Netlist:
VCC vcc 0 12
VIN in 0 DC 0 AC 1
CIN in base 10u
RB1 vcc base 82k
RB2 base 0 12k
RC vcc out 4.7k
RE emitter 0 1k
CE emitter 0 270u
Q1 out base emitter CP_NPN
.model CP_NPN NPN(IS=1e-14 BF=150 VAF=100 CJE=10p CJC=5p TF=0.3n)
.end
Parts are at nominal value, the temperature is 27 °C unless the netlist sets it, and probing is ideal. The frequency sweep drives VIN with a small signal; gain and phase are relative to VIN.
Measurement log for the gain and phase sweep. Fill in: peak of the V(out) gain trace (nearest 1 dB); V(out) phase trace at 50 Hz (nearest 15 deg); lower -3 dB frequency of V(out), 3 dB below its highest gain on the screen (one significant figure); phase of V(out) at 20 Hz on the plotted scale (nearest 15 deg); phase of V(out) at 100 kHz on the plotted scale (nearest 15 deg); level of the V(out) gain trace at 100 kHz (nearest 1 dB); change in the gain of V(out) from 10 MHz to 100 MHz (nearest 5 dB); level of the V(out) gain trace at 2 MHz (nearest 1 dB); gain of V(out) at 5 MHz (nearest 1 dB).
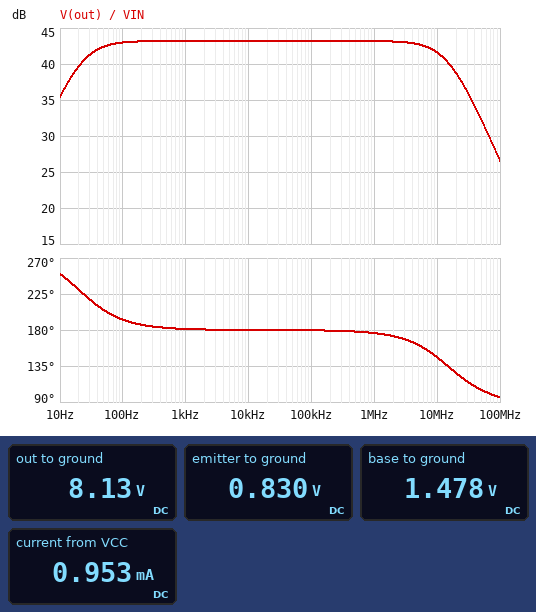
43 dB
210 deg
20 Hz
225 deg
180 deg
43 dB
-15 dB
43 dB
43 dB
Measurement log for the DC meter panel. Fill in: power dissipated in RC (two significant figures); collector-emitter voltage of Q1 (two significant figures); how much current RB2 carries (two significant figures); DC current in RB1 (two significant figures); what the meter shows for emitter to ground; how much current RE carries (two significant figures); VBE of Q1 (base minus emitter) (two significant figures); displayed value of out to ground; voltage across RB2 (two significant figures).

3.2 mW
7.3 V
120 µA
130 µA
0.830 V
830 µA
650 mV
8.13 V
1.5 V
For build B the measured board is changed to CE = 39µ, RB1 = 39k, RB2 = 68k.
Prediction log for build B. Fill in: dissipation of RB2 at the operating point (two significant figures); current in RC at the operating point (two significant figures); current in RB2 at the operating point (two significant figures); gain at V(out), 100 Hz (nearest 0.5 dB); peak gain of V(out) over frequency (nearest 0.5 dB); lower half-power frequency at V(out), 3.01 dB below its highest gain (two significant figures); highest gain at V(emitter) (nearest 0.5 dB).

130 µW
2.1 mA
43 µA
-4.0 dB
15.5 dB
940 Hz
-13.5 dB
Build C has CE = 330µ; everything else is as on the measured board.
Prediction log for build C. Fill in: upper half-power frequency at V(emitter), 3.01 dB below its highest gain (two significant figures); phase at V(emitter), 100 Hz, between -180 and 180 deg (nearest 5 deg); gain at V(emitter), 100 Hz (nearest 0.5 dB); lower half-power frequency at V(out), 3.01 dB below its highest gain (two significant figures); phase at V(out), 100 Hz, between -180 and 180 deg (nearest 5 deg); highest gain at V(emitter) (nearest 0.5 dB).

21 Hz
-80 deg
-16.5 dB
19 Hz
-170 deg
-2.5 dB
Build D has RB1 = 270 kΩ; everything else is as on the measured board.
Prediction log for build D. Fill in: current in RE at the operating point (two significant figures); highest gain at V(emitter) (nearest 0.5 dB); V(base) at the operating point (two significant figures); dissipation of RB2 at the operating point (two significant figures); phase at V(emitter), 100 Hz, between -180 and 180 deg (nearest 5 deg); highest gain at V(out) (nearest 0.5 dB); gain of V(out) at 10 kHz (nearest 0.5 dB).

3.6 µA
-28.0 dB
510 mV
22 µW
-90 deg
0 dB
-3.5 dB
